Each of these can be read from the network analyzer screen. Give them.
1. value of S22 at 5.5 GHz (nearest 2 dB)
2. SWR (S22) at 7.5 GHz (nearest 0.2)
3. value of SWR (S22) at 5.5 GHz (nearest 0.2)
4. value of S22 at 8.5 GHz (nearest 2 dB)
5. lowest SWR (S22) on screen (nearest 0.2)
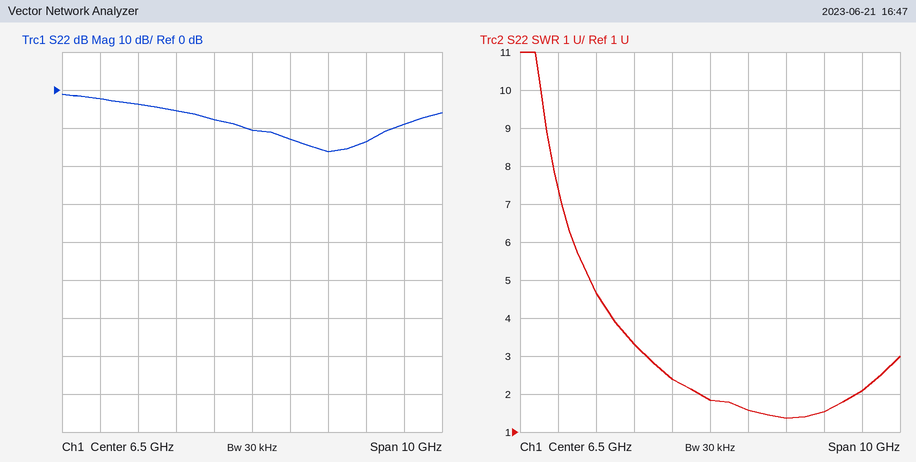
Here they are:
-8 dB
1.6
2.4
-16 dB
1.4
